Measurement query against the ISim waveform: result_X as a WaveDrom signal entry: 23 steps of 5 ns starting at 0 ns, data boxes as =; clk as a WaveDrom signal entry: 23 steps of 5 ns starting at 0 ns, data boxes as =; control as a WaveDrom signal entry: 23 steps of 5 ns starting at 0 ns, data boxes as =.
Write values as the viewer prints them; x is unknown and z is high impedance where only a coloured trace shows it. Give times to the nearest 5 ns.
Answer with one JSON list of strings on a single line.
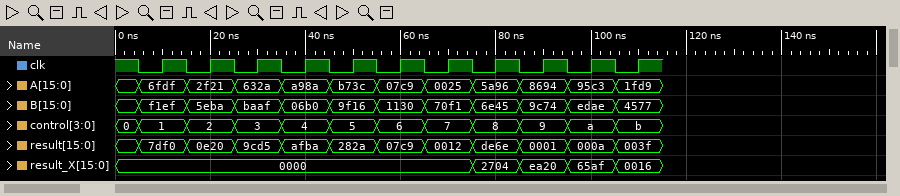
["{name: 'result_X', wave: '=..............=.=.=.=.', data: '0000 2704 ea20 65af 0016'}", "{name: 'clk', wave: '10101010101010101010101'}", "{name: 'control', wave: '==.=.=.=.=.=.=.=.=.=.=.', data: '0 1 2 3 4 5 6 7 8 9 a b'}"]
